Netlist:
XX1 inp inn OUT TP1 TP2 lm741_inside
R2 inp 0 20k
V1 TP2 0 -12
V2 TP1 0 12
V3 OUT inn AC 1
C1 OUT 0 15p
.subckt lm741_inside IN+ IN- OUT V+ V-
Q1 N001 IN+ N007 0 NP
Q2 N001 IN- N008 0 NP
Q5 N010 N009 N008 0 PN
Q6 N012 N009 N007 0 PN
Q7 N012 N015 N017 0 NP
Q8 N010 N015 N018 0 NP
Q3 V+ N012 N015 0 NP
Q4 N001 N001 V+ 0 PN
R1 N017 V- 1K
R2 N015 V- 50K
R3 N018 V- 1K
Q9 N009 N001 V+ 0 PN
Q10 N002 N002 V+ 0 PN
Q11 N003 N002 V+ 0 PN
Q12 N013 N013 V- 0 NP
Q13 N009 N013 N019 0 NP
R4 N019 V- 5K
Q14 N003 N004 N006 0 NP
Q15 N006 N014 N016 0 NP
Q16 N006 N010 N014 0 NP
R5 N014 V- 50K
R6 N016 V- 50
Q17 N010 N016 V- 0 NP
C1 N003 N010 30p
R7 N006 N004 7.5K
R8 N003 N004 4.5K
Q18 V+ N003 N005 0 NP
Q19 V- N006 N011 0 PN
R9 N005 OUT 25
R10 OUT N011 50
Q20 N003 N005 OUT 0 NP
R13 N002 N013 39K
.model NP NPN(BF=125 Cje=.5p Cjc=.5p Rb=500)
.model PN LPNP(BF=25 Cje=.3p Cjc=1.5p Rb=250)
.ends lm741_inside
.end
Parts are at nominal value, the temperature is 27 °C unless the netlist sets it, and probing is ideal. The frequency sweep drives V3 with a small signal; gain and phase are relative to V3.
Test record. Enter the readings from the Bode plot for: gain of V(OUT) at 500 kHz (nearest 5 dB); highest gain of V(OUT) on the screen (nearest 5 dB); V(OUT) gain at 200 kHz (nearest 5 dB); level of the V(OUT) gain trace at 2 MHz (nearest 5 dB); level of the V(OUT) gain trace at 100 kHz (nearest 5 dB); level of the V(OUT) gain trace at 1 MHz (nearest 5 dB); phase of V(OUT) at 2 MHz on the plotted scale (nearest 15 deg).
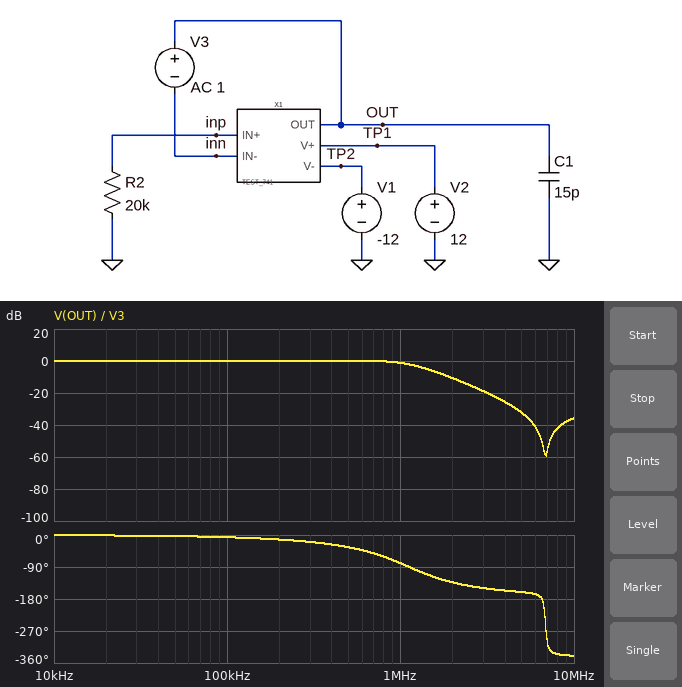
0 dB
0 dB
0 dB
-10 dB
0 dB
0 dB
-135 deg
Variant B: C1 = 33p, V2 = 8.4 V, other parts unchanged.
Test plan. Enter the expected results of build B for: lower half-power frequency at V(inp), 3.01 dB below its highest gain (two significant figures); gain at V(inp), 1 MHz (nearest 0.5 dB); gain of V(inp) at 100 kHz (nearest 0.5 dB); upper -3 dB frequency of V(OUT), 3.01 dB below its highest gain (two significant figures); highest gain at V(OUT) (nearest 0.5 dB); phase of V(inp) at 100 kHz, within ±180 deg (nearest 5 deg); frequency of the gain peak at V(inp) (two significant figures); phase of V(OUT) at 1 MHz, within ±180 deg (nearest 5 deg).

6.3 MHz
-28.0 dB
-55.5 dB
790 kHz
2.5 dB
-75 deg
13 MHz
-135 deg
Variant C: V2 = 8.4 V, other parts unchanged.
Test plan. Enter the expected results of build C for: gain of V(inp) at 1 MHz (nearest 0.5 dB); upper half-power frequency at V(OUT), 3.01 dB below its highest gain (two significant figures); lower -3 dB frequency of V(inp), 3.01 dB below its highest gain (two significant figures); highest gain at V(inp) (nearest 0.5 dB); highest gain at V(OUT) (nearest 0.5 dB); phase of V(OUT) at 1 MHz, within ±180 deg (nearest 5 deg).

-28.5 dB
1.1 MHz
6.2 MHz
-14.0 dB
0.5 dB
-90 deg
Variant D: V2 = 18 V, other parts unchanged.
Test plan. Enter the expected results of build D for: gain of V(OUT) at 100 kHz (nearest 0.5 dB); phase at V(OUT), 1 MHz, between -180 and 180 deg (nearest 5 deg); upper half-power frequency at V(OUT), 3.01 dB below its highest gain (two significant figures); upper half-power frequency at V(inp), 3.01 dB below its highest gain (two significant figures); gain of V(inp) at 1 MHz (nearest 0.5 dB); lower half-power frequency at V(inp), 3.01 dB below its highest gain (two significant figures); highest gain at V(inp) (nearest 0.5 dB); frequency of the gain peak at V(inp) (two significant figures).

0 dB
-65 deg
1.3 MHz
27 MHz
-30.5 dB
7.0 MHz
-13.0 dB
14 MHz
